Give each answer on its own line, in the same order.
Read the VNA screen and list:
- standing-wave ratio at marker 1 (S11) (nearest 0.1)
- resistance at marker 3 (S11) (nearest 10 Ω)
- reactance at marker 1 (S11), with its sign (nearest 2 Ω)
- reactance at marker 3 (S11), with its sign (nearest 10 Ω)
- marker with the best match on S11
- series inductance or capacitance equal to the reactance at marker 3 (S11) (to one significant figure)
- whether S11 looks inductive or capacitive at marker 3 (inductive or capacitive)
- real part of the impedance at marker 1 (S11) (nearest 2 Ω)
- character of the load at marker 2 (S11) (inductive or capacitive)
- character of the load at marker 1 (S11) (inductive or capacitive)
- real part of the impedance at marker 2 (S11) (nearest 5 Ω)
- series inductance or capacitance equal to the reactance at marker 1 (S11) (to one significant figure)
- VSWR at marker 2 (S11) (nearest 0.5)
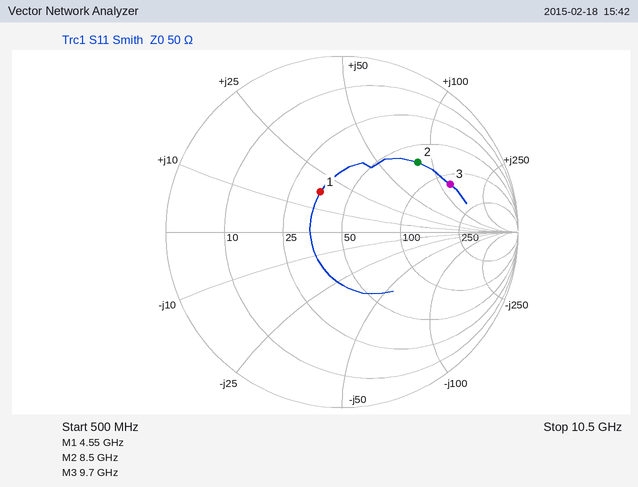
1.7
120 Ω
+18 Ω
+120 Ω
marker 1
2 nH
inductive
36 Ω
inductive
inductive
70 Ω
600 pH
4.0
